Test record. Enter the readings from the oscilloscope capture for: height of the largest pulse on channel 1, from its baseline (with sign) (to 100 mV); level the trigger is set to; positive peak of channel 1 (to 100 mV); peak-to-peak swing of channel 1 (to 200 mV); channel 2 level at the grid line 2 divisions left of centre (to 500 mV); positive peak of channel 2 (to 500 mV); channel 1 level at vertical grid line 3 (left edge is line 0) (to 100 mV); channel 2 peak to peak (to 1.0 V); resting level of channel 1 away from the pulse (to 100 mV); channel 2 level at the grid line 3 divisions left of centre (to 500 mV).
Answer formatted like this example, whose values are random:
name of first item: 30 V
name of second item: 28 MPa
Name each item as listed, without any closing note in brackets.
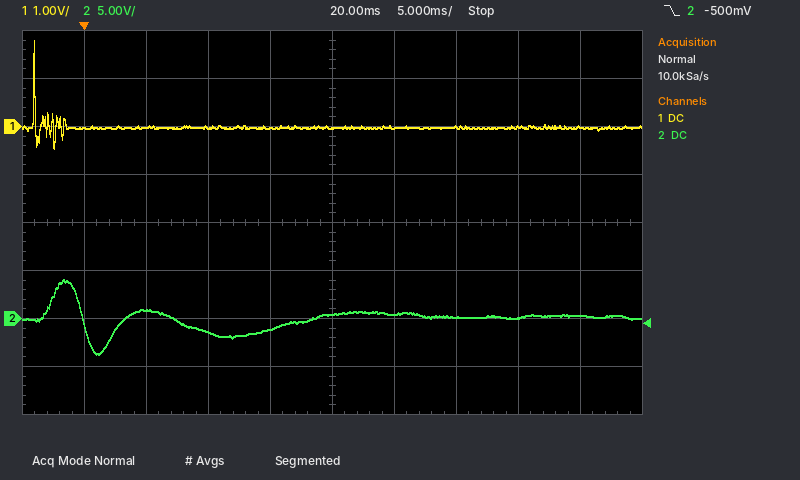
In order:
height of the largest pulse on channel 1, from its baseline (with sign): +1.8 V
level the trigger is set to: -500 mV
positive peak of channel 1: 1.8 V
peak-to-peak swing of channel 1: 2.2 V
channel 2 level at the grid line 2 divisions left of centre: -1.5 V
positive peak of channel 2: 4.0 V
channel 1 level at vertical grid line 3 (left edge is line 0): 0.0 V
channel 2 peak to peak: 8.0 V
resting level of channel 1 away from the pulse: 0.0 V
channel 2 level at the grid line 3 divisions left of centre: 1.0 V
